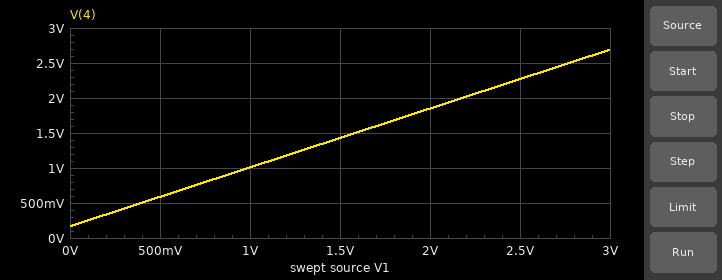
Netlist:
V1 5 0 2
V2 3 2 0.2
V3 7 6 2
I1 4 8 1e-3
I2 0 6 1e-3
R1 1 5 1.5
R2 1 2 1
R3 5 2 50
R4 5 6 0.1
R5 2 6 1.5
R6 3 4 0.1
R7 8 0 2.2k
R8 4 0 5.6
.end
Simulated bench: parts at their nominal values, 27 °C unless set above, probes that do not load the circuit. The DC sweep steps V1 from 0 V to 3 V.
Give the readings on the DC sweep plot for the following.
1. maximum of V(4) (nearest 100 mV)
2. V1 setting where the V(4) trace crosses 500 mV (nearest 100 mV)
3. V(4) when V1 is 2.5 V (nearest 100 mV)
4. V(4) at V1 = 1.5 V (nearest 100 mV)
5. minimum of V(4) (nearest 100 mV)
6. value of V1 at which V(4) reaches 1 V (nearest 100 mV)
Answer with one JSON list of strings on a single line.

["2.7 V", "400 mV", "2.3 V", "1.4 V", "200 mV", "1.0 V"]
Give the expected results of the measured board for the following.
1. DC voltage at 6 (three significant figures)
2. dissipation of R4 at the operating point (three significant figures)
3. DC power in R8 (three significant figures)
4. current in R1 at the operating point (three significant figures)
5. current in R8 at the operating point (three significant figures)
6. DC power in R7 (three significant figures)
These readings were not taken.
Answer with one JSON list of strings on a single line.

["1.98 V", "3.89 mW", "611 mW", "127 mA", "330 mA", "2.20 mW"]
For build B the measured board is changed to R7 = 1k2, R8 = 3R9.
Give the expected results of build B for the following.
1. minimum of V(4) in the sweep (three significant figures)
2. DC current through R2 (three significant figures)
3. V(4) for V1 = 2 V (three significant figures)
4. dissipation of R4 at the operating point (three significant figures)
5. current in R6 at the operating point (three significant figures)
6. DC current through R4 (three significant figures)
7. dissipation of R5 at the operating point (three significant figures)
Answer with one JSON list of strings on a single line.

["157 mV", "170 mA", "1.73 V", "7.02 mW", "445 mA", "265 mA", "106 mW"]
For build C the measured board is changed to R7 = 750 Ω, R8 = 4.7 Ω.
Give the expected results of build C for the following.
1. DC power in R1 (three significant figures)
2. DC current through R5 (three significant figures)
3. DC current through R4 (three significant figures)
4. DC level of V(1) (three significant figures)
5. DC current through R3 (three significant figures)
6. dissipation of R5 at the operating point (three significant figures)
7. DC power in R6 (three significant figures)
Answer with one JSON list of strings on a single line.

["32.2 mW", "229 mA", "228 mA", "1.78 V", "7.33 mA", "78.7 mW", "14.7 mW"]
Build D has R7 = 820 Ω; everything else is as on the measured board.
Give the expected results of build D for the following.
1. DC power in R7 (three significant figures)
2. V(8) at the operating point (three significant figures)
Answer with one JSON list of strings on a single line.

["820 µW", "820 mV"]
